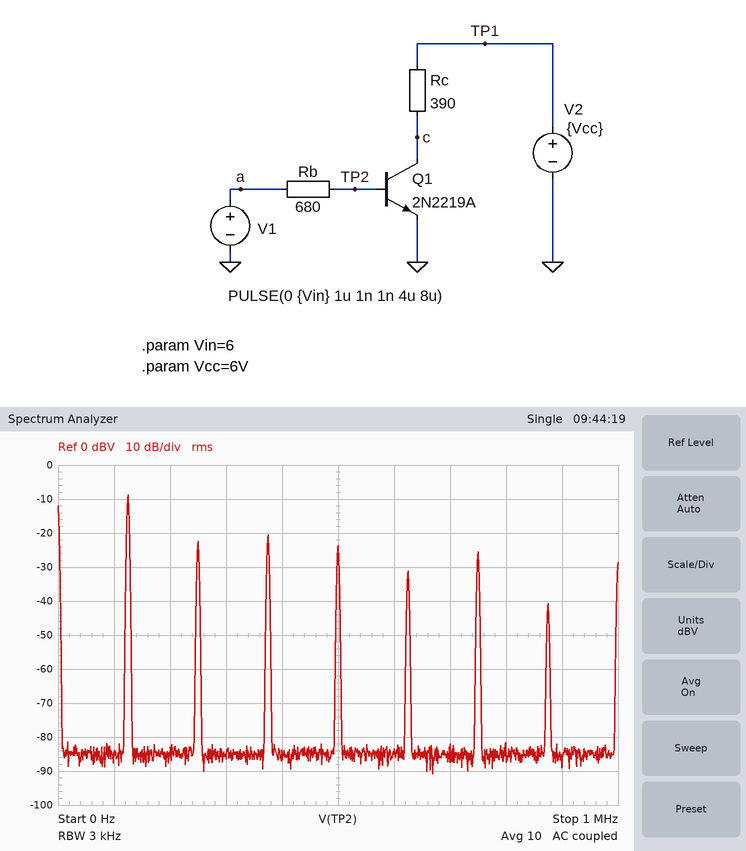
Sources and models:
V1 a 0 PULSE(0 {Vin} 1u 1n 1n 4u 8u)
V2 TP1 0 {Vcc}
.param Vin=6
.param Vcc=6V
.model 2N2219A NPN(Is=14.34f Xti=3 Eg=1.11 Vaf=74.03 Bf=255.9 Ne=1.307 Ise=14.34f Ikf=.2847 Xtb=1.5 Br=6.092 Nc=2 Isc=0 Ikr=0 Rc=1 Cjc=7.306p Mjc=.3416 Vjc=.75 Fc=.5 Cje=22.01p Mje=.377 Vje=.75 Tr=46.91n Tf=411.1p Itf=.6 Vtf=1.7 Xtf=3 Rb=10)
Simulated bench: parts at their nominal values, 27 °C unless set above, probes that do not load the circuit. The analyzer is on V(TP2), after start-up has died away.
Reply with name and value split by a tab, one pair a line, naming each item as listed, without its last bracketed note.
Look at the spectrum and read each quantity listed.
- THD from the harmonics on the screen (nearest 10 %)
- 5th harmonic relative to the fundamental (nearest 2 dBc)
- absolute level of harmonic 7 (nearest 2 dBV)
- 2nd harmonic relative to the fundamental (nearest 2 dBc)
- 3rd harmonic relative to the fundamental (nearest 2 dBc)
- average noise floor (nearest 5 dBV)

THD from the harmonics on the screen	40 %
5th harmonic relative to the fundamental	-22 dBc
absolute level of harmonic 7	-40 dBV
2nd harmonic relative to the fundamental	-14 dBc
3rd harmonic relative to the fundamental	-12 dBc
average noise floor	-85 dBV
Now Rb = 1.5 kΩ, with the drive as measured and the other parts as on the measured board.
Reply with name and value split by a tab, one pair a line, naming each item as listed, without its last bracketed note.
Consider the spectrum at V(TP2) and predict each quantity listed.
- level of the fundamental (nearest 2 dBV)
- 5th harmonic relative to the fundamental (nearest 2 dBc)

level of the fundamental	-10 dBV
5th harmonic relative to the fundamental	-24 dBc
